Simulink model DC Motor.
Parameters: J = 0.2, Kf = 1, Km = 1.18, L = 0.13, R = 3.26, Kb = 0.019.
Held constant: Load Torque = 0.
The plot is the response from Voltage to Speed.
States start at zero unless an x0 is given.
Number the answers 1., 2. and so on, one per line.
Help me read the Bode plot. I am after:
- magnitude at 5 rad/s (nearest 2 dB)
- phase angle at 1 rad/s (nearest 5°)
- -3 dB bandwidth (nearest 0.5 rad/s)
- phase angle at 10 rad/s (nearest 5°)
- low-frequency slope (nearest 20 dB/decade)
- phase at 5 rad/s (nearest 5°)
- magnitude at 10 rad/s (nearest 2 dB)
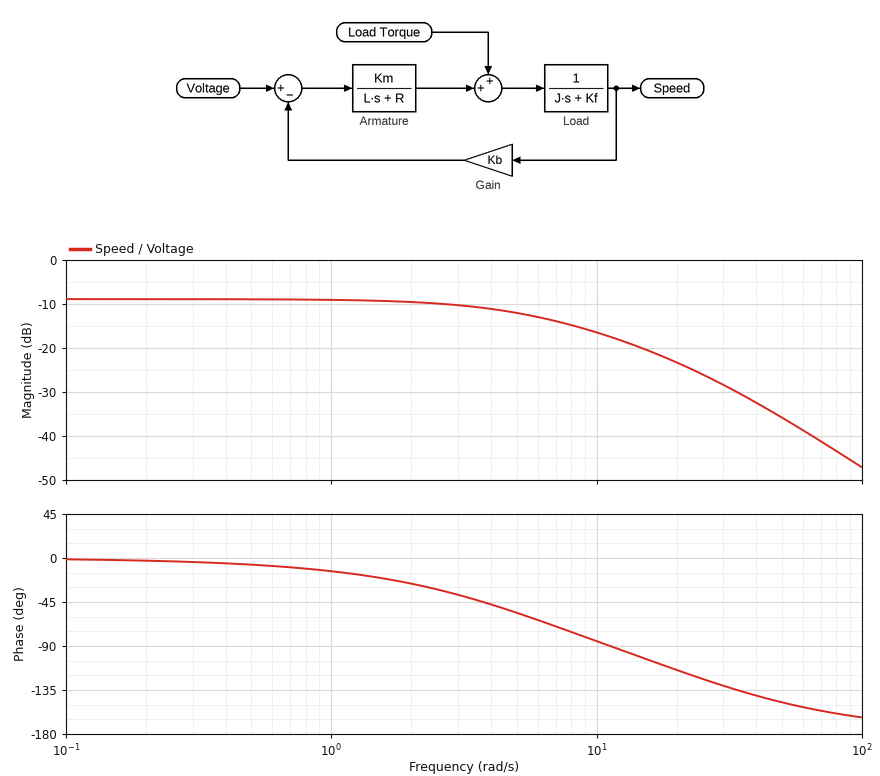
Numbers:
1. -12 dB
2. -15°
3. 5.0 rad/s
4. -85°
5. 0 dB/decade
6. -55°
7. -16 dB
